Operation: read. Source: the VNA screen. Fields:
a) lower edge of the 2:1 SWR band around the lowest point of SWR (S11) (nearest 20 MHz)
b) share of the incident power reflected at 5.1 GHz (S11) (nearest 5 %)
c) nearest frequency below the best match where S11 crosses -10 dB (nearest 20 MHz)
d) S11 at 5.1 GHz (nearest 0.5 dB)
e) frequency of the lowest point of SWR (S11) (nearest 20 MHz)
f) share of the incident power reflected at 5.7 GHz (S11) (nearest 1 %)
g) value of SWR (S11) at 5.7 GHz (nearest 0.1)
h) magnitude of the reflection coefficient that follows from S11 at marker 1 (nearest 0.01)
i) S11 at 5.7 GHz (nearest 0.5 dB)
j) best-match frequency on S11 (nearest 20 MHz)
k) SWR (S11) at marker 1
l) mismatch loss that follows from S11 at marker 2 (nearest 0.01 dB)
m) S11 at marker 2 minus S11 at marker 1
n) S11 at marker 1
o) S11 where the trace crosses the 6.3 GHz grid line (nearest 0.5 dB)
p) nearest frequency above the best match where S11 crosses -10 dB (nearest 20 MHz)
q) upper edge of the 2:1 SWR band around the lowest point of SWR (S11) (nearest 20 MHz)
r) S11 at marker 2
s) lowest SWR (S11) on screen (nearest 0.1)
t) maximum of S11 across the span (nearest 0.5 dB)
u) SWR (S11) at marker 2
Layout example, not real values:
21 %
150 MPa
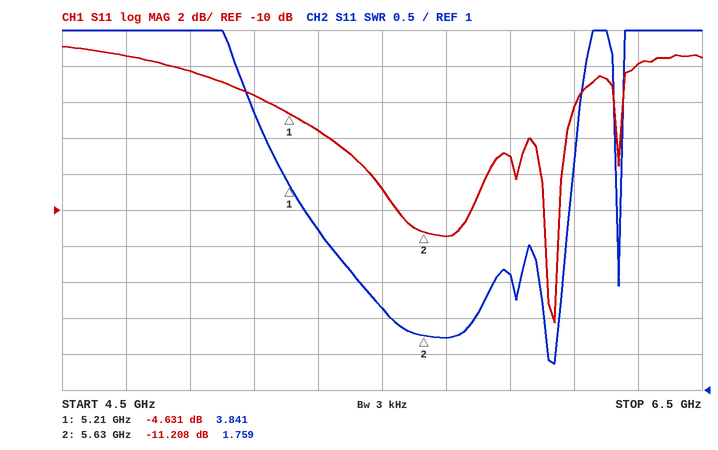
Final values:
6.00 GHz
45 %
6.00 GHz
-3.5 dB
6.04 GHz
7 %
1.7
0.59
-11.5 dB
6.04 GHz
3.841
0.34 dB
-6.577 dB
-4.631 dB
-2.0 dB
6.06 GHz
6.06 GHz
-11.208 dB
1.4
-1.0 dB
1.759
